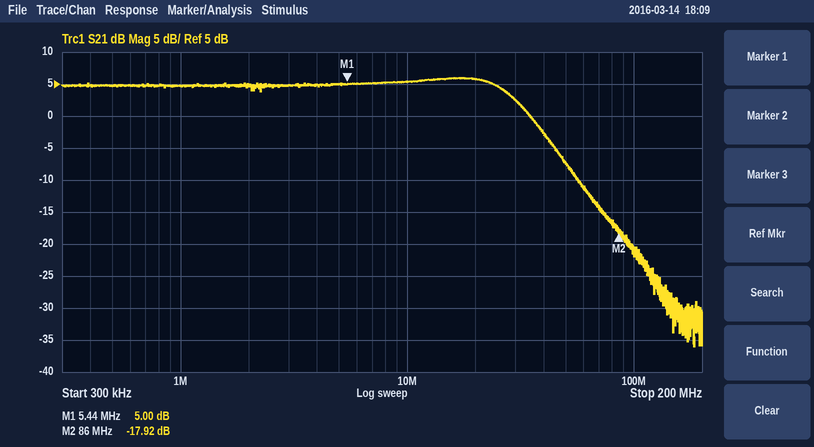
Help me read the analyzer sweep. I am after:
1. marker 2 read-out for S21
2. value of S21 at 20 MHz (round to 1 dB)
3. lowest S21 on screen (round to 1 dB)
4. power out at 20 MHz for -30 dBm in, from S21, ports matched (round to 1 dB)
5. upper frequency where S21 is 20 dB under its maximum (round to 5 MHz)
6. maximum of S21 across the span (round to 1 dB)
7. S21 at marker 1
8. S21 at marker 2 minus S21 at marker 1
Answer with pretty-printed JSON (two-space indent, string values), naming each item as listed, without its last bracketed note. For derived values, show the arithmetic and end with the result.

{
  "marker 2 read-out for S21": "-17.92 dB",
  "value of S21 at 20 MHz": "6 dB",
  "lowest S21 on screen": "-36 dB",
  "power out at 20 MHz for -30 dBm in, from S21, ports matched": "-30 dBm + (6 dB) = -24 dBm",
  "upper frequency where S21 is 20 dB under its maximum": "70 MHz",
  "maximum of S21 across the span": "6 dB",
  "S21 at marker 1": "5.00 dB",
  "S21 at marker 2 minus S21 at marker 1": "-17.92 − (5) = -22.92 dB"
}
